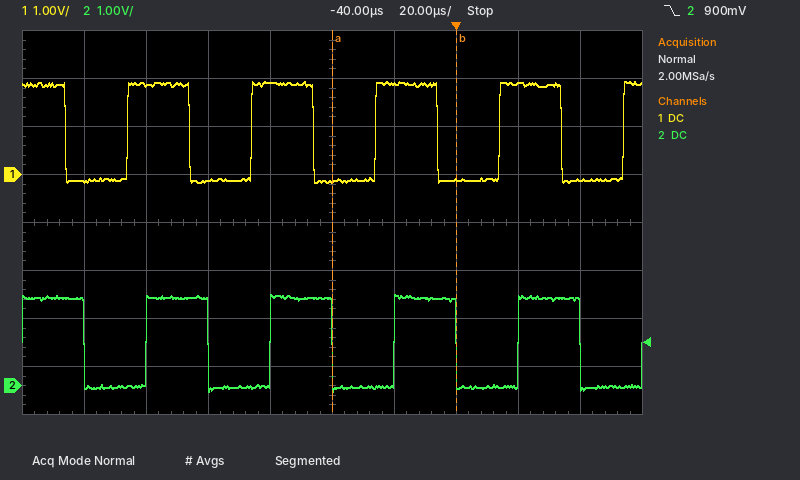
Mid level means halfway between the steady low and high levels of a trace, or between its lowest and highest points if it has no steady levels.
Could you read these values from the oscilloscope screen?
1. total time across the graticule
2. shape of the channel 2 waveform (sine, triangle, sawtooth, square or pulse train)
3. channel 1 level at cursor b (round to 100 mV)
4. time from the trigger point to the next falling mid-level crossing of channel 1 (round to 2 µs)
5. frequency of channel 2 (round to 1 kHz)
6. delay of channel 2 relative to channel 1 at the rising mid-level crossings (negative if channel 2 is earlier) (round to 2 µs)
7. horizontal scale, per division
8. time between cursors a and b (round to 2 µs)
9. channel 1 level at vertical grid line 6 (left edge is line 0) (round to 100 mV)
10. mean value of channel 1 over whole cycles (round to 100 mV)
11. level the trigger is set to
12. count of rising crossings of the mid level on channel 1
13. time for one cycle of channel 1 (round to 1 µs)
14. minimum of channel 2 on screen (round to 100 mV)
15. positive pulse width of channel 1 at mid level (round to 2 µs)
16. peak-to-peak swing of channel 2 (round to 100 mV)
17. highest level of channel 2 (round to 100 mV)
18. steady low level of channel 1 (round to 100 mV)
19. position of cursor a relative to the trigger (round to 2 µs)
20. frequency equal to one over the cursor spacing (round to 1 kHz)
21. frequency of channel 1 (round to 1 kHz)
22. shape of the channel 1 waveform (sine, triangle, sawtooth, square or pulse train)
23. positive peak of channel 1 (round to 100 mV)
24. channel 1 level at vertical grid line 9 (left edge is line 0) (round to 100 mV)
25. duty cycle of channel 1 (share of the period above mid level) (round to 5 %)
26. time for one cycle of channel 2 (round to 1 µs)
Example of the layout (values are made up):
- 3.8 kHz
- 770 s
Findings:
- 200 µs
- square
- -100 mV
- 34 µs
- 25 kHz
- +6 µs
- 20 µs
- 40 µs
- 1.9 V
- 900 mV
- 900 mV
- 5
- 40 µs
- -100 mV
- 20 µs
- 2.0 V
- 1.9 V
- -100 mV
- -40 µs
- 25 kHz
- 25 kHz
- square
- 1.9 V
- -100 mV
- 50 %
- 40 µs
